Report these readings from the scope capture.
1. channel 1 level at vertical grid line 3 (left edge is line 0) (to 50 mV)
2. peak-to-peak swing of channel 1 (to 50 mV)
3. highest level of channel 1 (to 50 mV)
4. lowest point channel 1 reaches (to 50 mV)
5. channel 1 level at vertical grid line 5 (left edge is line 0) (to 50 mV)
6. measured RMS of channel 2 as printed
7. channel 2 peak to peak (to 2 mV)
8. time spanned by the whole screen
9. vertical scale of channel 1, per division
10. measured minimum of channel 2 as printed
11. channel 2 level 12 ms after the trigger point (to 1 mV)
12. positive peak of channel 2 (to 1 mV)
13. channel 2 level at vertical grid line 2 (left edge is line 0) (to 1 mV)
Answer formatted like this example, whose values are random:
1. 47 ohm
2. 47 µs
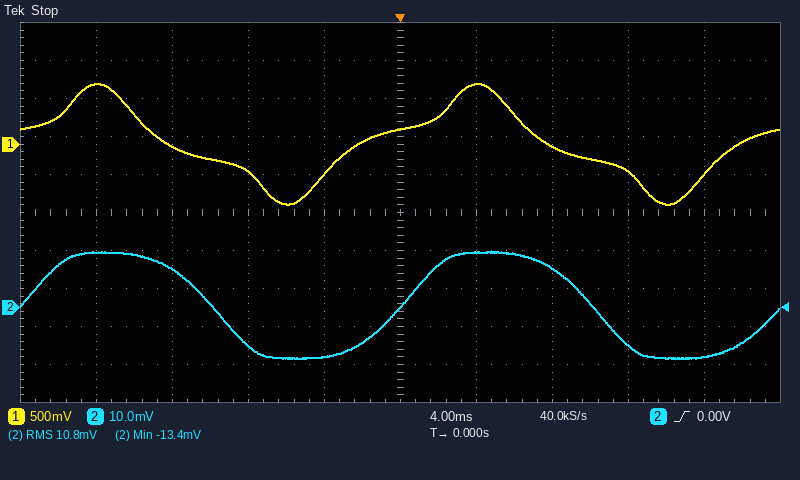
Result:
1. -350 mV
2. 1.60 V
3. 800 mV
4. -800 mV
5. 200 mV
6. 10.8 mV
7. 28 mV
8. 40 ms
9. 500 mV
10. -13.4 mV
11. -10 mV
12. 15 mV
13. 10 mV
